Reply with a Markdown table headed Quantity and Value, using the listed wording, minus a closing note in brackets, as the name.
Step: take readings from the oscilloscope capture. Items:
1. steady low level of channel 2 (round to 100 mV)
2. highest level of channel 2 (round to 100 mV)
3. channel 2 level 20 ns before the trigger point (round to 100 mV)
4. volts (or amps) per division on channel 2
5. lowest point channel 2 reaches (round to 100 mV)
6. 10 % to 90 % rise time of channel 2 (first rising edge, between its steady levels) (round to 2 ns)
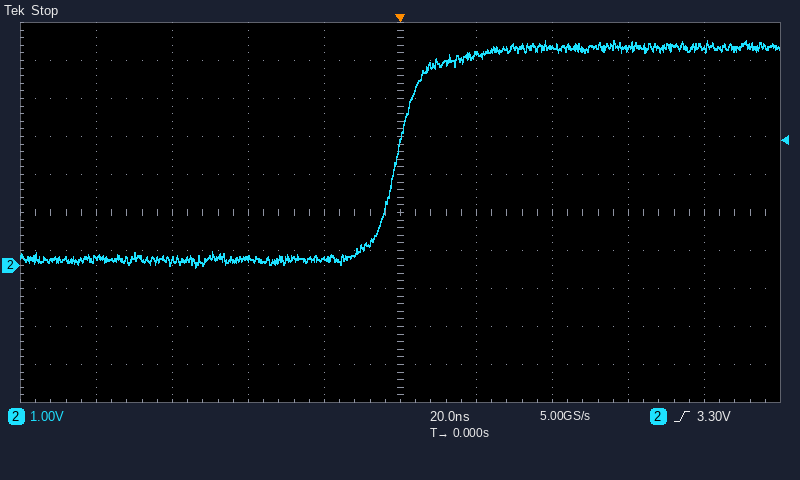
| Quantity | Value |
|---|---|
| steady low level of channel 2 | 200 mV |
| highest level of channel 2 | 5.9 V |
| channel 2 level 20 ns before the trigger point | 200 mV |
| volts (or amps) per division on channel 2 | 1 V |
| lowest point channel 2 reaches | 0.0 V |
| 10 % to 90 % rise time of channel 2 (first rising edge, between its steady levels) | 14 ns |
